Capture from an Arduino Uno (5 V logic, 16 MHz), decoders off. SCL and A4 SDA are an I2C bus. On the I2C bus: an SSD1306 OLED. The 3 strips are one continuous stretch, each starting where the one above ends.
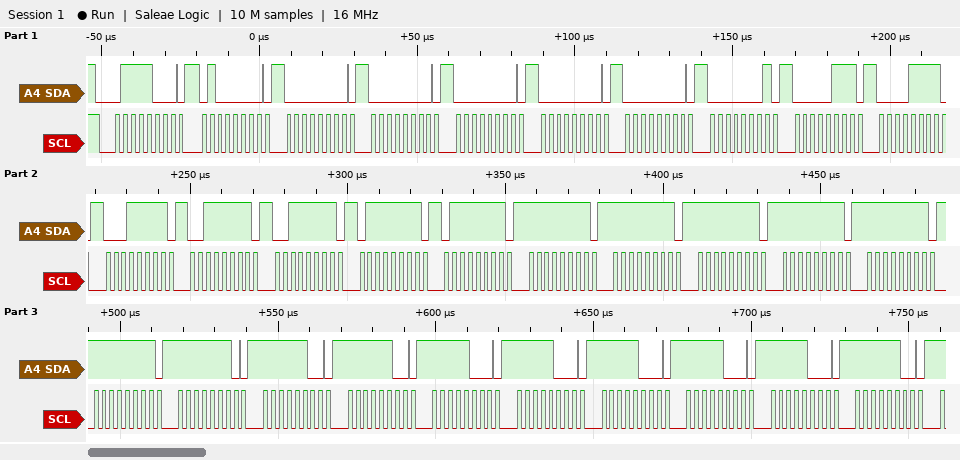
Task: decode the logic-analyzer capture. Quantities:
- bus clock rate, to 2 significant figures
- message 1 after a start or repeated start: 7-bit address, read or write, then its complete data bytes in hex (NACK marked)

400 kHz
0x3C write: 40 00 00 00 00 00 01 07 0F 1F 3F 3F 7F 7F FF FF FF FF FF FF FE FC FC F8 F8 F8 F8 F8 FC
